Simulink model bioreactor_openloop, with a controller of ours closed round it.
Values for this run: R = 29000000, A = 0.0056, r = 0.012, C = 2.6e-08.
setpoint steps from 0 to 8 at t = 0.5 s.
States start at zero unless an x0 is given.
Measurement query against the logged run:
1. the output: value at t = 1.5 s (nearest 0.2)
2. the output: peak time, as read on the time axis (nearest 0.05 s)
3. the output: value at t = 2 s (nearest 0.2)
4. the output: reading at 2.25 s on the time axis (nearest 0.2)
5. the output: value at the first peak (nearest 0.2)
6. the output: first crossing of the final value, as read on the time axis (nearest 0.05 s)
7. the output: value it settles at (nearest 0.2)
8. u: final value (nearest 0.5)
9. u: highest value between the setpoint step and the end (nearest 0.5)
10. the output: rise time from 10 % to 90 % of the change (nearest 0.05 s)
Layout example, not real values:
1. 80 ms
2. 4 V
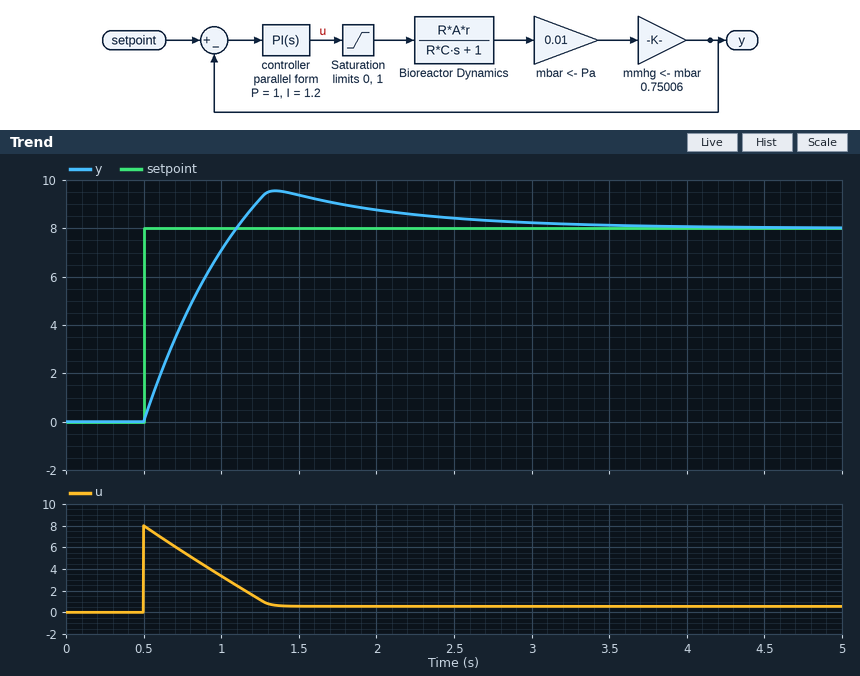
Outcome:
1. 9.4
2. 1.35 s
3. 8.8
4. 8.6
5. 9.6
6. 1.10 s
7. 8.0
8. 0.5
9. 8.0
10. 0.45 s
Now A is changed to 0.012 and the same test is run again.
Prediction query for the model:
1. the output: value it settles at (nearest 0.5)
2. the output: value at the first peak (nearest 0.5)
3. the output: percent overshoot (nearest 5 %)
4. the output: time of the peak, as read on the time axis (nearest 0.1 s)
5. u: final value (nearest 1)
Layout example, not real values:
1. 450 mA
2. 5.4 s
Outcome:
1. 8.0
2. 8.5
3. 10 %
4. 0.8 s
5. 0
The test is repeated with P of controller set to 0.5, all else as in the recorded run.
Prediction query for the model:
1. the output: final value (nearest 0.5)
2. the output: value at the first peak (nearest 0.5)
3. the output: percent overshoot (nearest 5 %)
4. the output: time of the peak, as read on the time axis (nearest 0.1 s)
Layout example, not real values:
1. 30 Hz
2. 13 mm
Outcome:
1. 8.0
2. 10.5
3. 30 %
4. 1.5 s
